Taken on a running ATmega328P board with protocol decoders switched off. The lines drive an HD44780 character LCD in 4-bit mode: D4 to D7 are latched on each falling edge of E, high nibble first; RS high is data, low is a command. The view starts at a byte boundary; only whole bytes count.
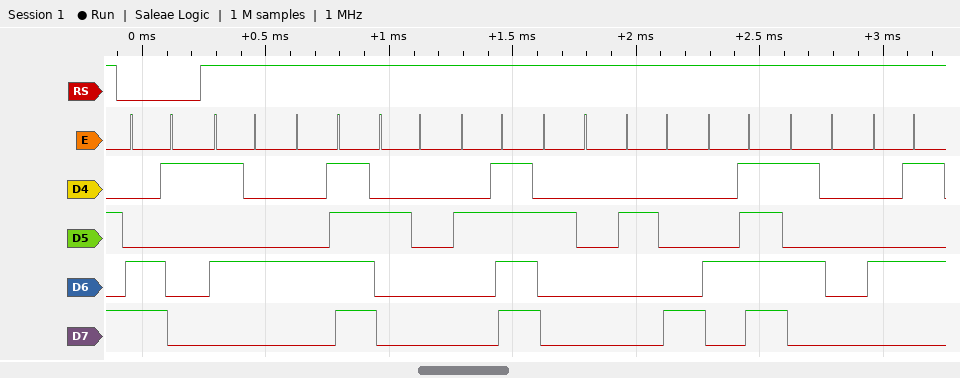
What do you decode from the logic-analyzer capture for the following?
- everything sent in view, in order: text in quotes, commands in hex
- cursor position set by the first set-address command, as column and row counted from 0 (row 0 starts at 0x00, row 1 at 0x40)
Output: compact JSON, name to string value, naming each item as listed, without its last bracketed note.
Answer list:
{"everything sent in view, in order: text in quotes, commands in hex": "0xC1 \"TO / (OPE\"", "cursor position set by the first set-address command, as column and row counted from 0": "column 1, row 1"}
